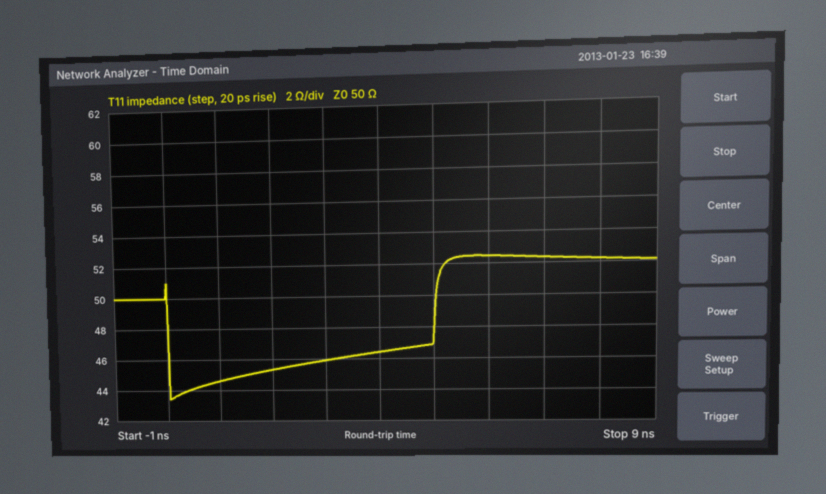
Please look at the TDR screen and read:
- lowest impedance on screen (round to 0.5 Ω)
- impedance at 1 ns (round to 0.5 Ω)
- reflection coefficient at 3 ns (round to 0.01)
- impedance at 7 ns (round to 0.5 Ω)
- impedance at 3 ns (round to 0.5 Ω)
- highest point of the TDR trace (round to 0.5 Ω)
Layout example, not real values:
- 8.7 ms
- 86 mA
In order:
- 43.5 Ω
- 44.5 Ω
- -0.04
- 52.5 Ω
- 46.0 Ω
- 52.5 Ω
